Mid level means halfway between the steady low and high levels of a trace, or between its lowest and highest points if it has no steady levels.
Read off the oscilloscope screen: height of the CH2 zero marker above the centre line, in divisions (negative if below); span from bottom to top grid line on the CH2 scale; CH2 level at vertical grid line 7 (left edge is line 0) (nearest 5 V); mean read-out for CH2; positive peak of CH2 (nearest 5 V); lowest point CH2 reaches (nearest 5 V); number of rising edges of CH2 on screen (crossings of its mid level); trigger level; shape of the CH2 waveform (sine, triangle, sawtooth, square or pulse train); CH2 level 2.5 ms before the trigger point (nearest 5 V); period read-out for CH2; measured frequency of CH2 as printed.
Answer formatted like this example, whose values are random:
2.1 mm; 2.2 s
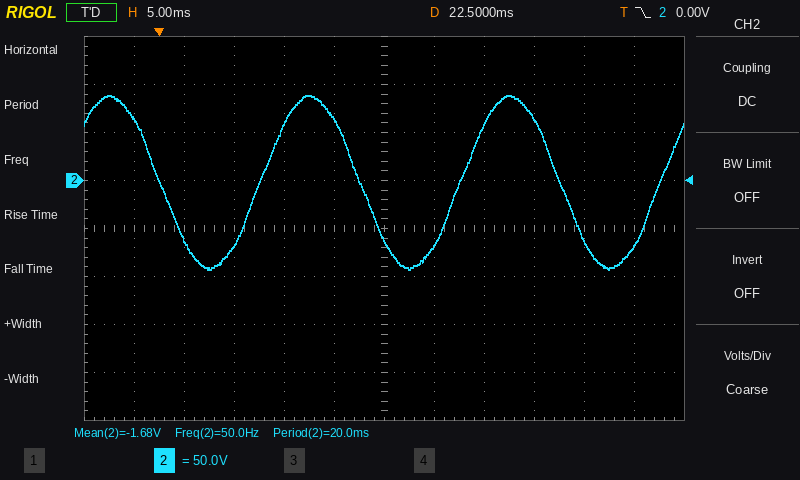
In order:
+1.0 div; 400 V; -65 V; -1.68 V; 90 V; -95 V; 3; 0.00 V; sine; 65 V; 20.0 ms; 50.0 Hz
